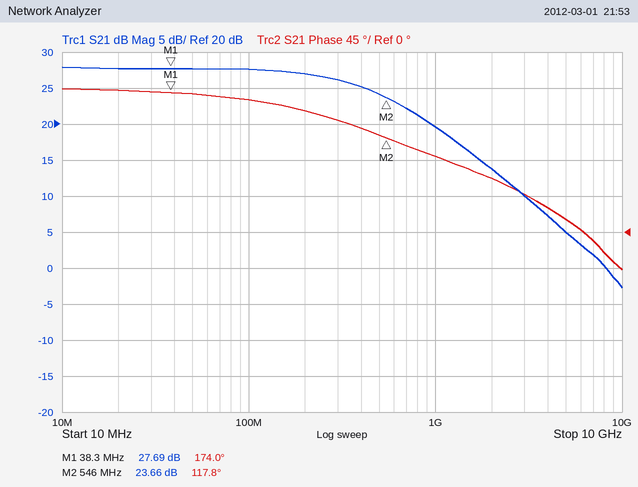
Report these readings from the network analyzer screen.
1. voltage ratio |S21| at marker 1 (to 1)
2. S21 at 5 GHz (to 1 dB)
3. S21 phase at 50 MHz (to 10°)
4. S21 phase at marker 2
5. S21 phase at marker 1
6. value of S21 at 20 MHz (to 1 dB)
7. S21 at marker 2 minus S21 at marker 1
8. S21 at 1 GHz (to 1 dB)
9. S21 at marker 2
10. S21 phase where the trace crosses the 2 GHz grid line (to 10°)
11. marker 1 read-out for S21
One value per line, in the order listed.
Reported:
24
5 dB
170°
117.8°
174.0°
28 dB
-4.03 dB
20 dB
23.66 dB
70°
27.69 dB
